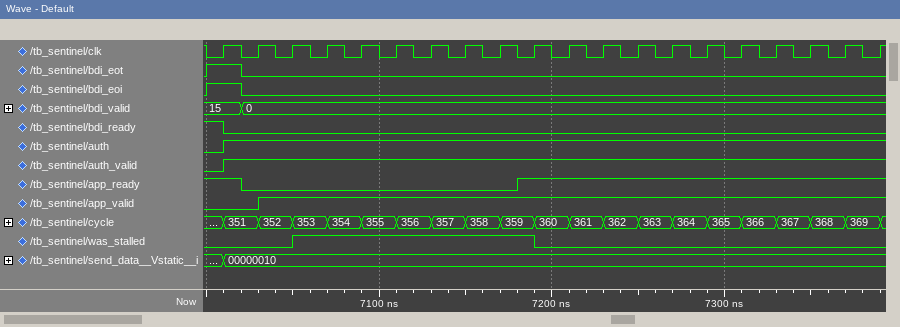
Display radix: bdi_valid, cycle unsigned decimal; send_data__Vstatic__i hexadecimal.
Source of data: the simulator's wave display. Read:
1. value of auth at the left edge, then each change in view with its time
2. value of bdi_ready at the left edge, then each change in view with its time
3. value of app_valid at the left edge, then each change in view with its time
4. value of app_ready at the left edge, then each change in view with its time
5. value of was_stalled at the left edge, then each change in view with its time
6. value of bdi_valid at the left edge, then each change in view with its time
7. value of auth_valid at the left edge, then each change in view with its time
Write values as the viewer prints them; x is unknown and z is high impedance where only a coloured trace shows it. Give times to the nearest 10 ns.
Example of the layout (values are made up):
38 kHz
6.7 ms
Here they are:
0, 1 at 7010 ns
1, 0 at 7010 ns
0, 1 at 7030 ns
1, 0 at 7020 ns, 1 at 7180 ns
0, 1 at 7050 ns, 0 at 7190 ns
15, 0 at 7020 ns
0, 1 at 7010 ns
